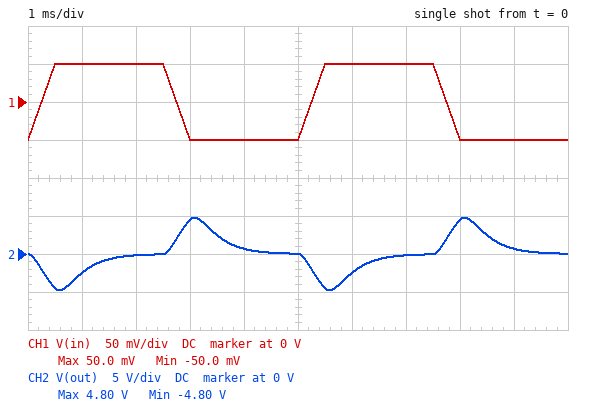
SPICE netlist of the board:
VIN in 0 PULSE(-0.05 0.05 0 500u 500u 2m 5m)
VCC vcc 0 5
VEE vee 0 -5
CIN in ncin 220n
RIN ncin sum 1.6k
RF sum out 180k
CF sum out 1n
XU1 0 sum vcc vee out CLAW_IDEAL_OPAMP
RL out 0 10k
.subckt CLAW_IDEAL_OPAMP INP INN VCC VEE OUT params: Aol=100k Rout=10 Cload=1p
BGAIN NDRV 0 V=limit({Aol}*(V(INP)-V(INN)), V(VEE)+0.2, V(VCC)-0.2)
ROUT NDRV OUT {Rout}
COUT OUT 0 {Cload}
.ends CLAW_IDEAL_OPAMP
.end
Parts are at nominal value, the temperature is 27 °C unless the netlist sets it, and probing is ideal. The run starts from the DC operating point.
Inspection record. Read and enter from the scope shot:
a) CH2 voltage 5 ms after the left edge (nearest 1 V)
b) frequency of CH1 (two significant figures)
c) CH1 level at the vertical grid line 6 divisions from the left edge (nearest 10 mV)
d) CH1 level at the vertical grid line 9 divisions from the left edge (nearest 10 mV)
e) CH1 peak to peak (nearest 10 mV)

0 V
200 Hz
50 mV
-50 mV
100 mV
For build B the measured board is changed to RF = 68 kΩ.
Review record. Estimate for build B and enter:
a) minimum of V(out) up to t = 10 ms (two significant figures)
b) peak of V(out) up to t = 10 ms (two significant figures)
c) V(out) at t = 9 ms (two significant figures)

-2.1 V
2.1 V
160 mV
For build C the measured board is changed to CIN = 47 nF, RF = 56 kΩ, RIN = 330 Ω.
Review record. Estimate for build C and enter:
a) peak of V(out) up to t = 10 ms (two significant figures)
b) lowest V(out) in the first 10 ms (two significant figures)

530 mV
-530 mV
